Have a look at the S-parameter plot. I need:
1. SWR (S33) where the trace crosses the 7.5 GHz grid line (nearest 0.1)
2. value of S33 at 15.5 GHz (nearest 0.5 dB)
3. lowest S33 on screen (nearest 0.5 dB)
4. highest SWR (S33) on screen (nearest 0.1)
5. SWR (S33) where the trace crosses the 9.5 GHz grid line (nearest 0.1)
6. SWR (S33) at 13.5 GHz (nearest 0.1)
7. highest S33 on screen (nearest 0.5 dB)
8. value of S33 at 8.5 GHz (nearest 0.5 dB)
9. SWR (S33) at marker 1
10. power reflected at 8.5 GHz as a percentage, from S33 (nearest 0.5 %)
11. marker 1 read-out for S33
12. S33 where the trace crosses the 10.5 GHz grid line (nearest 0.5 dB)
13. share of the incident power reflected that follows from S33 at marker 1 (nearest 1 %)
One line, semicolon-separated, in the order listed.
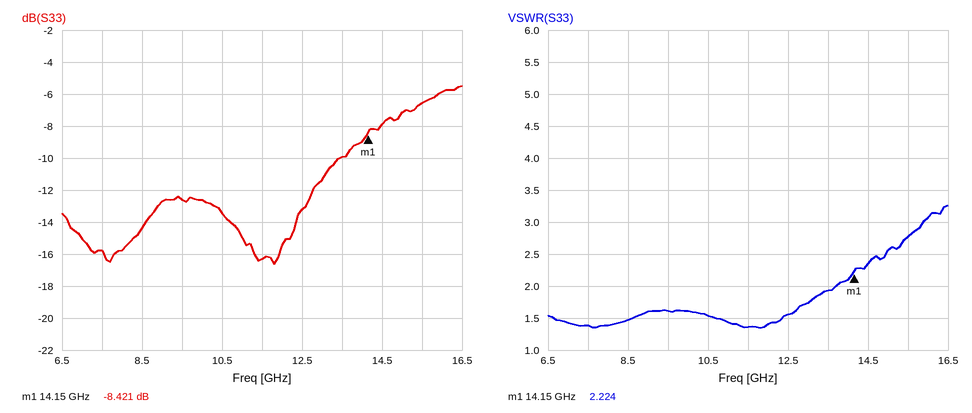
1.4; -6.5 dB; -16.5 dB; 3.3; 1.6; 1.9; -5.5 dB; -14.5 dB; 2.224; 3.5 %; -8.421 dB; -13.5 dB; 14 %
